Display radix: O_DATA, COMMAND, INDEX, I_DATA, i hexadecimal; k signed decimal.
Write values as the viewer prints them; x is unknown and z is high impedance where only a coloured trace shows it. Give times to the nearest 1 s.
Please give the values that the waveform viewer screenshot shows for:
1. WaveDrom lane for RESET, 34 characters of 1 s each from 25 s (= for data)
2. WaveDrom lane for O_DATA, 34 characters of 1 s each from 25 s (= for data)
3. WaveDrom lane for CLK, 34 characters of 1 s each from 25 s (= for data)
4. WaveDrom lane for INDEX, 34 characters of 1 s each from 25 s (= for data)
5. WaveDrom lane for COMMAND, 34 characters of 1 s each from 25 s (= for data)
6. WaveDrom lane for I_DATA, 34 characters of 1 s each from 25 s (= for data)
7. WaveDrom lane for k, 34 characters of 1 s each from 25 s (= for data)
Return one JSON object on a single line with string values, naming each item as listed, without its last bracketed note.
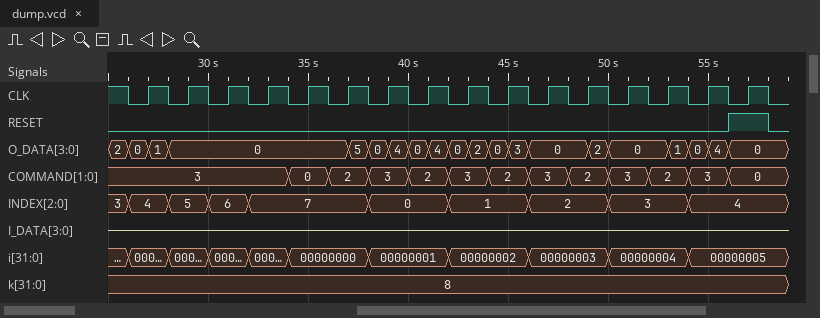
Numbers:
{"WaveDrom lane for RESET, 34 characters of 1 s each from 25 s": "{name: 'RESET', wave: '0..............................1.0'}", "WaveDrom lane for O_DATA, 34 characters of 1 s each from 25 s": "{name: 'O_DATA', wave: '====........==========..==..====..', data: '2 0 1 0 5 0 4 0 4 0 2 0 3 0 2 0 1 0 4 0'}", "WaveDrom lane for CLK, 34 characters of 1 s each from 25 s": "{name: 'CLK', wave: '1010101010101010101010101010101010'}", "WaveDrom lane for INDEX, 34 characters of 1 s each from 25 s": "{name: 'INDEX', wave: '==.=.=.=.....=...=...=...=...=....', data: '3 4 5 6 7 0 1 2 3 4'}", "WaveDrom lane for COMMAND, 34 characters of 1 s each from 25 s": "{name: 'COMMAND', wave: '=........=.=.=.=.=.=.=.=.=.=.=.=..', data: '3 0 2 3 2 3 2 3 2 3 2 3 0'}", "WaveDrom lane for I_DATA, 34 characters of 1 s each from 25 s": "{name: 'I_DATA', wave: 'z.................................'}", "WaveDrom lane for k, 34 characters of 1 s each from 25 s": "{name: 'k', wave: '=.................................', data: '8'}"}
